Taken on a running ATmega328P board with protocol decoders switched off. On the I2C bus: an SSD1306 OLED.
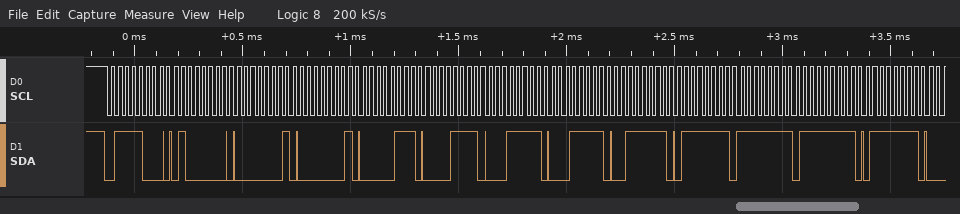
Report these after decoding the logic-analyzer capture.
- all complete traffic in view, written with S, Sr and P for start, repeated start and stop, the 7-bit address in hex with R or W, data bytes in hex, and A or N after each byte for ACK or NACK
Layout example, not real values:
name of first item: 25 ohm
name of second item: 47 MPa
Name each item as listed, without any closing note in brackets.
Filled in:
all complete traffic in view, written with S, Sr and P for start, repeated start and stop, the 7-bit address in hex with R or W, data bytes in hex, and A or N after each byte for ACK or NACK: S 3CW A 40 A 01 A 01 A 07 A 0F A 1F A 1F A 3F A 7F A FF A FF A 7F A
